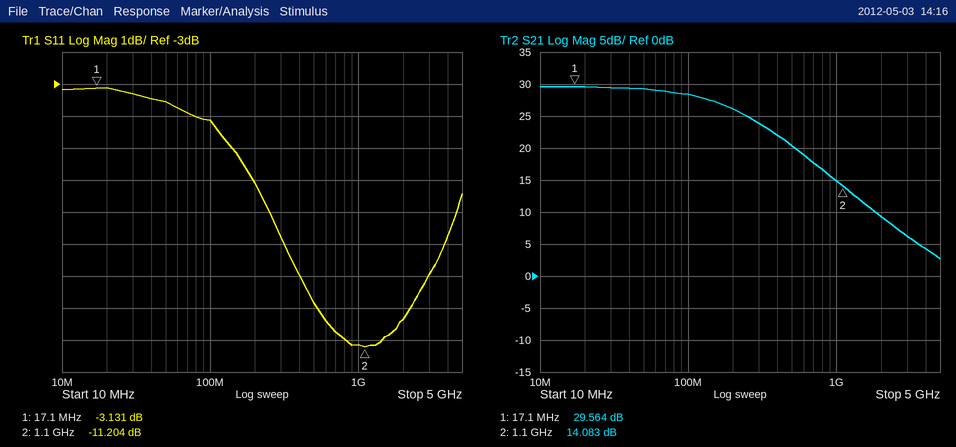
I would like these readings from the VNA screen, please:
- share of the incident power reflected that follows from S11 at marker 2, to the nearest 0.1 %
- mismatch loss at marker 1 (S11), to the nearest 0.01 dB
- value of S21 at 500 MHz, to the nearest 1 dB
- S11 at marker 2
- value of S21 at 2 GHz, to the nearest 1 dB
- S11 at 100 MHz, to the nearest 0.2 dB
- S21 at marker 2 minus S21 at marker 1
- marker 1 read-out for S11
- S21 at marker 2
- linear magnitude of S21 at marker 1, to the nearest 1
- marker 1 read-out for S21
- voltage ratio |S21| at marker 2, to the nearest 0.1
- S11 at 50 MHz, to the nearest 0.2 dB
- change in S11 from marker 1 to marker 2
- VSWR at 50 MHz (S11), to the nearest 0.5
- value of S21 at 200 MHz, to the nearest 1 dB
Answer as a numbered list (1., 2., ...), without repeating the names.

1. 7.6 %
2. 2.89 dB
3. 20 dB
4. -11.204 dB
5. 9 dB
6. -4.2 dB
7. -15.481 dB
8. -3.131 dB
9. 14.083 dB
10. 30
11. 29.564 dB
12. 5.1
13. -3.6 dB
14. -8.073 dB
15. 5.0
16. 26 dB
